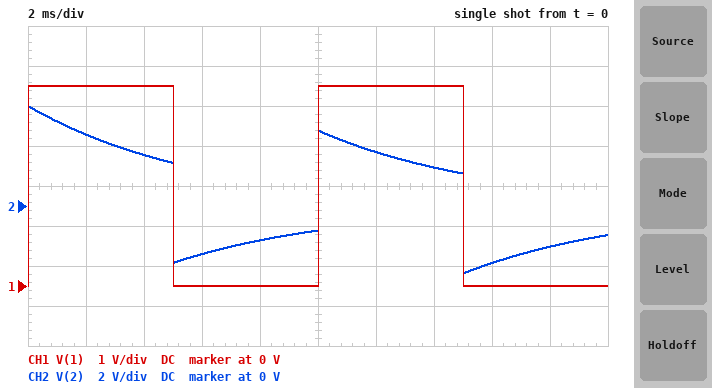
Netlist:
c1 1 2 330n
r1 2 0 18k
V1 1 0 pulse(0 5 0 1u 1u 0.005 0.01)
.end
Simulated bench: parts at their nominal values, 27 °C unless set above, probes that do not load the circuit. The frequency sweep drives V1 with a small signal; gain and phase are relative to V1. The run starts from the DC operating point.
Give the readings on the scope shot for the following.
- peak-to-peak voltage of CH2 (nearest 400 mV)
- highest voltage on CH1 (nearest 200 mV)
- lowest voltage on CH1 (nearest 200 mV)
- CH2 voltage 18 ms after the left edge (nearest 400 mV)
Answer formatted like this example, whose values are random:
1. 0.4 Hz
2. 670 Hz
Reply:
1. 8.4 V
2. 5.0 V
3. 0 V
4. -2.0 V
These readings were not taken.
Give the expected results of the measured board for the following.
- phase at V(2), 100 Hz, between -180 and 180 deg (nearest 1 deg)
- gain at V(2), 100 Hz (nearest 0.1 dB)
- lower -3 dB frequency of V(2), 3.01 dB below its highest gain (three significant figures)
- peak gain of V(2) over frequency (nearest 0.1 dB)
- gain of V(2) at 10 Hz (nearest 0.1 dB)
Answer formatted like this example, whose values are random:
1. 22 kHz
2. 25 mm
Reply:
1. 15 deg
2. -0.3 dB
3. 26.8 Hz
4. 0 dB
5. -9.1 dB
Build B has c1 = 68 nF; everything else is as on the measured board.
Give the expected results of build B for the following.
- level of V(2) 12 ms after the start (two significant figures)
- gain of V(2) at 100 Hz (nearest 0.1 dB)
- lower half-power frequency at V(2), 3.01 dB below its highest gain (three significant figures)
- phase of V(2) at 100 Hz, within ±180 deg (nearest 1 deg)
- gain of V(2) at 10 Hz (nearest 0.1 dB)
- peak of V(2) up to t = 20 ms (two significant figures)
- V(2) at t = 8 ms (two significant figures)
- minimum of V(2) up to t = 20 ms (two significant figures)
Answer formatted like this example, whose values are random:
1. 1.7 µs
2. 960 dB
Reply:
1. 960 mV
2. -4.3 dB
3. 130 Hz
4. 52 deg
5. -22.3 dB
6. 5.0 V
7. -420 mV
8. -4.9 V
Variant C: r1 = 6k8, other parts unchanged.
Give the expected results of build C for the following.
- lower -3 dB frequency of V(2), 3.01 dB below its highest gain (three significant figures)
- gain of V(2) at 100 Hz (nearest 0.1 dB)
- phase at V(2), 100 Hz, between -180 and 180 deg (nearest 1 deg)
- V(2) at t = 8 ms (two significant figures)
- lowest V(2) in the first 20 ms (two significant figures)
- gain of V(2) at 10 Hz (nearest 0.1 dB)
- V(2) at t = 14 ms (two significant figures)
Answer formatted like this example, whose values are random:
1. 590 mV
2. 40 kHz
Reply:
1. 70.9 Hz
2. -1.8 dB
3. 35 deg
4. -1.2 V
5. -4.5 V
6. -17.1 dB
7. 760 mV
